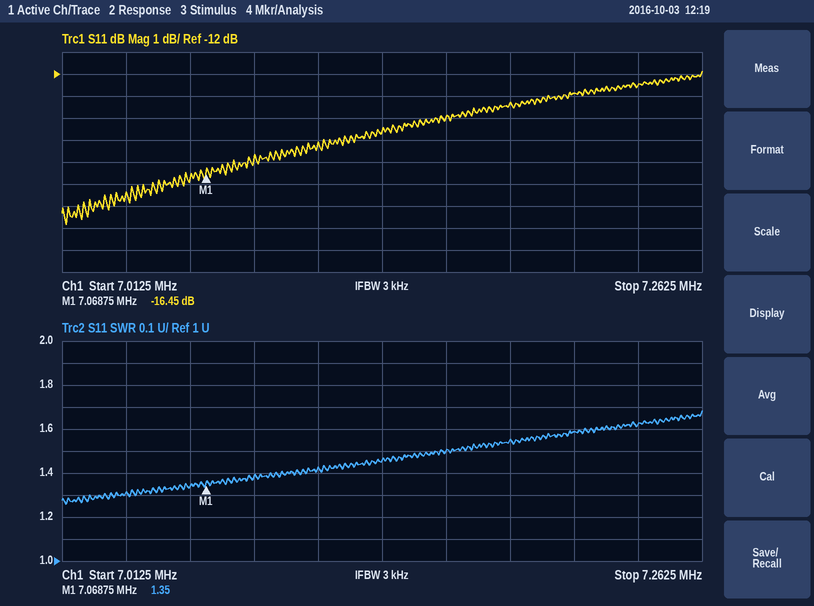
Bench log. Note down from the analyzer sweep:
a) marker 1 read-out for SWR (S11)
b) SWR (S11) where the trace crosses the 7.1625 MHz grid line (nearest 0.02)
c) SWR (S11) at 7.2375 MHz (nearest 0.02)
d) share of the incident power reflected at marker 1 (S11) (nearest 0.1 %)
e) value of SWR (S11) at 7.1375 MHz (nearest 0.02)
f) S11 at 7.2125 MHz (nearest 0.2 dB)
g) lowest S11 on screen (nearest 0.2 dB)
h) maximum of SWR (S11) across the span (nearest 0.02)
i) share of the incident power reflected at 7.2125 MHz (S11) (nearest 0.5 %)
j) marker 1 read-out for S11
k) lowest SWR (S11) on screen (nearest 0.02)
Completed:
1.35
1.50
1.62
2.3 %
1.46
-12.8 dB
-18.8 dB
1.68
5.0 %
-16.45 dB
1.26
